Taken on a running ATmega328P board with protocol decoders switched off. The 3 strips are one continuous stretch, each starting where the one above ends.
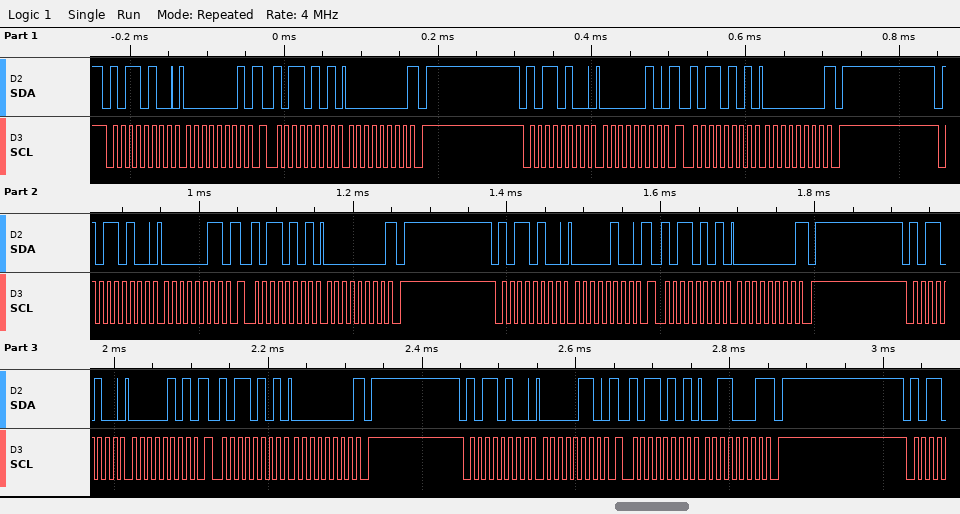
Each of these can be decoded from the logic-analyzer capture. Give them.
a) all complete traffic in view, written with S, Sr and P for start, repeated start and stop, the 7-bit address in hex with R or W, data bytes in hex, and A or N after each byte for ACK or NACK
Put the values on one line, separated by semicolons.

S 5AW A 01 A Sr 5AR A 00 N P S 5AW A 02 A Sr 5AR A 00 N P S 5AW A 03 A Sr 5AR A 00 N P S 5AW A 04 A Sr 5AR A 00 N P S 5AW A 05 A Sr 5AR A 00 N P S 5AW A 06 A Sr 5AR A 31 N P
